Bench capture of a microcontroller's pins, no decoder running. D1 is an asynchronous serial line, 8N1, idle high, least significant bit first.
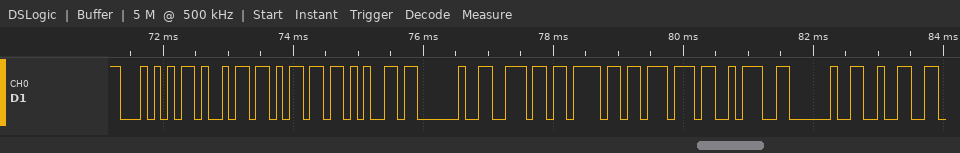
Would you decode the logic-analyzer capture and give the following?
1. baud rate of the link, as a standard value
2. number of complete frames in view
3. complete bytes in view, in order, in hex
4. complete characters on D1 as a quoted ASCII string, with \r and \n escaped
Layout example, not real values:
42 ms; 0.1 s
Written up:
9600 baud; 11; 0x54 0x69 0x6D 0x65 0x20 0x6E 0x6F 0x77 0x3A 0x20 0x32; "Time now: 2"
